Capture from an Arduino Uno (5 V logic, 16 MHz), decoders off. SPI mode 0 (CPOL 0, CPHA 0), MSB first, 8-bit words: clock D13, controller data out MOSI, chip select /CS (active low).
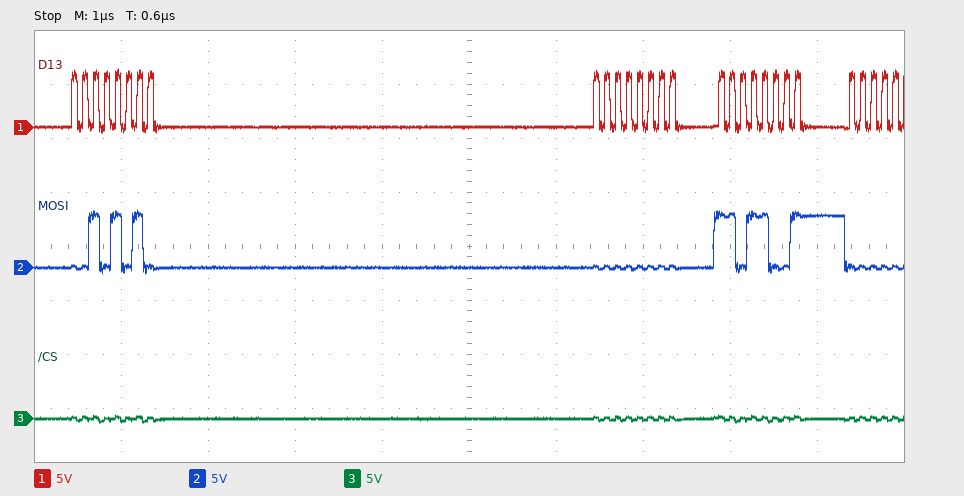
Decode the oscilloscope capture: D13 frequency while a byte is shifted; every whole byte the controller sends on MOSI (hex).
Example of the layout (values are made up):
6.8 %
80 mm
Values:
8 MHz
2A 00 D9
